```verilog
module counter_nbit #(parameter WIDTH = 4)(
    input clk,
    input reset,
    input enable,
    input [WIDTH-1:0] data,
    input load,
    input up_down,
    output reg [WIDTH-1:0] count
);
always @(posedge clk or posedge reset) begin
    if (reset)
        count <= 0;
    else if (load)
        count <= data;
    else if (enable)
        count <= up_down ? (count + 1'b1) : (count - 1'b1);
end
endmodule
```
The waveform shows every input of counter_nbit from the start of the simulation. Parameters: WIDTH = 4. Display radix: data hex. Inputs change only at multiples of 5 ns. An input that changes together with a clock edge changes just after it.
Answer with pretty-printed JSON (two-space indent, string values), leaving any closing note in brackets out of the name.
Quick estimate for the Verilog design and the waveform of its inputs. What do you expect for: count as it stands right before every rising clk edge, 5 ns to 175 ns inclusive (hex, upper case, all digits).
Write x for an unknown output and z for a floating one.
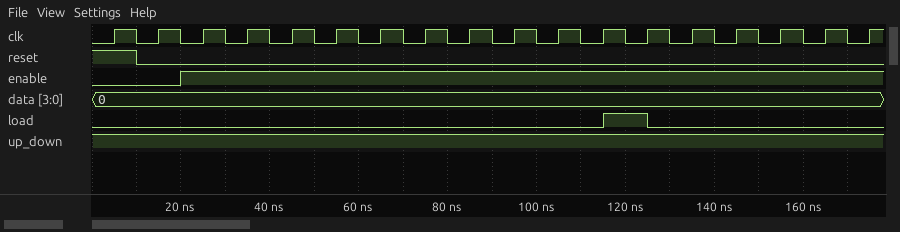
{
  "count as it stands right before every rising clk edge, 5 ns to 175 ns inclusive": "0, 0, 0, 1, 2, 3, 4, 5, 6, 7, 8, 9, A, 0, 1, 2, 3, 4"
}
